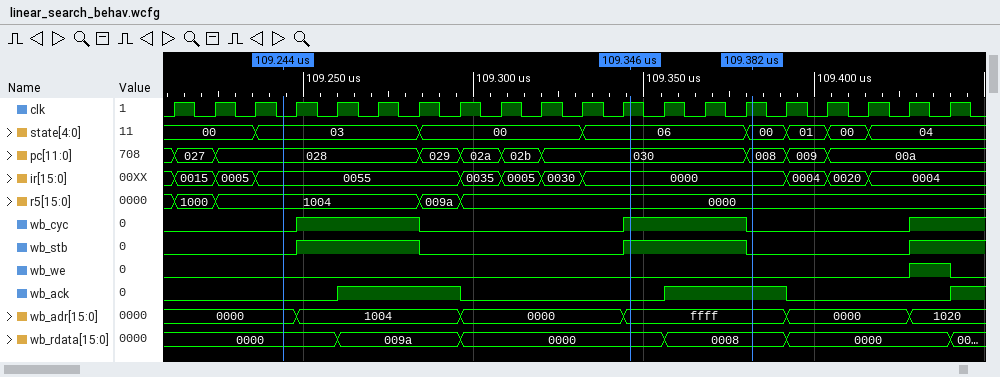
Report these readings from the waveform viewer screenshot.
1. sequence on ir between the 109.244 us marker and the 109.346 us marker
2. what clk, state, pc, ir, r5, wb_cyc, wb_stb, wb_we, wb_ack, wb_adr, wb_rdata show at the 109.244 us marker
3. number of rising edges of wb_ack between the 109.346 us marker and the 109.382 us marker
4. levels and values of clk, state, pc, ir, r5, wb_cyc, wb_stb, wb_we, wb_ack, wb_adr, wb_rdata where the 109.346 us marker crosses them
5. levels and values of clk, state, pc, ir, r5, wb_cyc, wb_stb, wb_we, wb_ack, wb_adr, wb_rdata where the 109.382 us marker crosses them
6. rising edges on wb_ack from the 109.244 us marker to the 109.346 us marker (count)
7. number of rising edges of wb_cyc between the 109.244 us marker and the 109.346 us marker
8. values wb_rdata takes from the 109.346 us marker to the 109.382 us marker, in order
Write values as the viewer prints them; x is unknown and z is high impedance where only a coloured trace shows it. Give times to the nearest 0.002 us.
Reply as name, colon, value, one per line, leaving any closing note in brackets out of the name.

sequence on ir between the 109.244 us marker and the 109.346 us marker: 0055, 0035, 0005, 0030, 0000
what clk, state, pc, ir, r5, wb_cyc, wb_stb, wb_we, wb_ack, wb_adr, wb_rdata show at the 109.244 us marker: clk=0, state=03, pc=028, ir=0055, r5=1004, wb_cyc=0, wb_stb=0, wb_we=0, wb_ack=0, wb_adr=0000, wb_rdata=0000
number of rising edges of wb_ack between the 109.346 us marker and the 109.382 us marker: 1
levels and values of clk, state, pc, ir, r5, wb_cyc, wb_stb, wb_we, wb_ack, wb_adr, wb_rdata where the 109.346 us marker crosses them: clk=1, state=06, pc=030, ir=0000, r5=0000, wb_cyc=1, wb_stb=1, wb_we=0, wb_ack=0, wb_adr=ffff, wb_rdata=0000
levels and values of clk, state, pc, ir, r5, wb_cyc, wb_stb, wb_we, wb_ack, wb_adr, wb_rdata where the 109.382 us marker crosses them: clk=1, state=00, pc=008, ir=0000, r5=0000, wb_cyc=0, wb_stb=0, wb_we=0, wb_ack=1, wb_adr=ffff, wb_rdata=0008
rising edges on wb_ack from the 109.244 us marker to the 109.346 us marker: 1
number of rising edges of wb_cyc between the 109.244 us marker and the 109.346 us marker: 2
values wb_rdata takes from the 109.346 us marker to the 109.382 us marker, in order: 0000, 0008
